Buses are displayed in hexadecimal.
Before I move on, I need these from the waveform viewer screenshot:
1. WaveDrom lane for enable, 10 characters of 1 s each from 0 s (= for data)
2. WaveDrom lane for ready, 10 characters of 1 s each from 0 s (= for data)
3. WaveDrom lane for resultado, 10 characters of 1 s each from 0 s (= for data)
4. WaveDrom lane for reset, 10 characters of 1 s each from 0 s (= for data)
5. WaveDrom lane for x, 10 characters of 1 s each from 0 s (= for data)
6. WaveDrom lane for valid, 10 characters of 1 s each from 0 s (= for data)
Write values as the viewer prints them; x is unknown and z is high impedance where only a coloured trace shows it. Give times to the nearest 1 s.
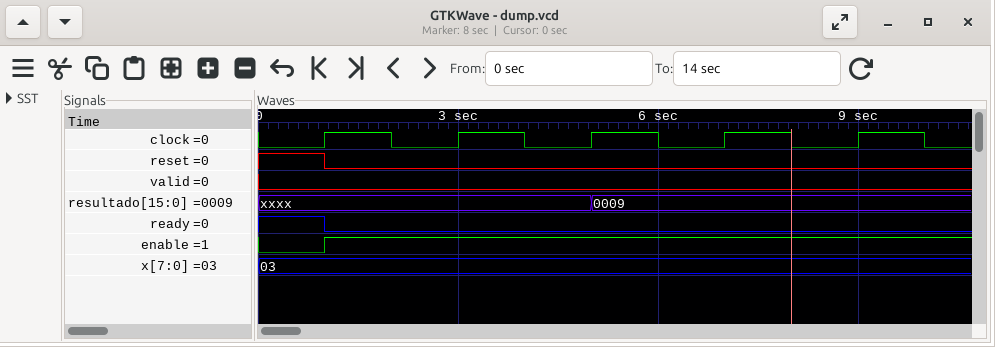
{name: 'enable', wave: '01........'}
{name: 'ready', wave: '10........'}
{name: 'resultado', wave: 'x....=....', data: '0009'}
{name: 'reset', wave: '10........'}
{name: 'x', wave: '=.........', data: '03'}
{name: 'valid', wave: '0.........'}
